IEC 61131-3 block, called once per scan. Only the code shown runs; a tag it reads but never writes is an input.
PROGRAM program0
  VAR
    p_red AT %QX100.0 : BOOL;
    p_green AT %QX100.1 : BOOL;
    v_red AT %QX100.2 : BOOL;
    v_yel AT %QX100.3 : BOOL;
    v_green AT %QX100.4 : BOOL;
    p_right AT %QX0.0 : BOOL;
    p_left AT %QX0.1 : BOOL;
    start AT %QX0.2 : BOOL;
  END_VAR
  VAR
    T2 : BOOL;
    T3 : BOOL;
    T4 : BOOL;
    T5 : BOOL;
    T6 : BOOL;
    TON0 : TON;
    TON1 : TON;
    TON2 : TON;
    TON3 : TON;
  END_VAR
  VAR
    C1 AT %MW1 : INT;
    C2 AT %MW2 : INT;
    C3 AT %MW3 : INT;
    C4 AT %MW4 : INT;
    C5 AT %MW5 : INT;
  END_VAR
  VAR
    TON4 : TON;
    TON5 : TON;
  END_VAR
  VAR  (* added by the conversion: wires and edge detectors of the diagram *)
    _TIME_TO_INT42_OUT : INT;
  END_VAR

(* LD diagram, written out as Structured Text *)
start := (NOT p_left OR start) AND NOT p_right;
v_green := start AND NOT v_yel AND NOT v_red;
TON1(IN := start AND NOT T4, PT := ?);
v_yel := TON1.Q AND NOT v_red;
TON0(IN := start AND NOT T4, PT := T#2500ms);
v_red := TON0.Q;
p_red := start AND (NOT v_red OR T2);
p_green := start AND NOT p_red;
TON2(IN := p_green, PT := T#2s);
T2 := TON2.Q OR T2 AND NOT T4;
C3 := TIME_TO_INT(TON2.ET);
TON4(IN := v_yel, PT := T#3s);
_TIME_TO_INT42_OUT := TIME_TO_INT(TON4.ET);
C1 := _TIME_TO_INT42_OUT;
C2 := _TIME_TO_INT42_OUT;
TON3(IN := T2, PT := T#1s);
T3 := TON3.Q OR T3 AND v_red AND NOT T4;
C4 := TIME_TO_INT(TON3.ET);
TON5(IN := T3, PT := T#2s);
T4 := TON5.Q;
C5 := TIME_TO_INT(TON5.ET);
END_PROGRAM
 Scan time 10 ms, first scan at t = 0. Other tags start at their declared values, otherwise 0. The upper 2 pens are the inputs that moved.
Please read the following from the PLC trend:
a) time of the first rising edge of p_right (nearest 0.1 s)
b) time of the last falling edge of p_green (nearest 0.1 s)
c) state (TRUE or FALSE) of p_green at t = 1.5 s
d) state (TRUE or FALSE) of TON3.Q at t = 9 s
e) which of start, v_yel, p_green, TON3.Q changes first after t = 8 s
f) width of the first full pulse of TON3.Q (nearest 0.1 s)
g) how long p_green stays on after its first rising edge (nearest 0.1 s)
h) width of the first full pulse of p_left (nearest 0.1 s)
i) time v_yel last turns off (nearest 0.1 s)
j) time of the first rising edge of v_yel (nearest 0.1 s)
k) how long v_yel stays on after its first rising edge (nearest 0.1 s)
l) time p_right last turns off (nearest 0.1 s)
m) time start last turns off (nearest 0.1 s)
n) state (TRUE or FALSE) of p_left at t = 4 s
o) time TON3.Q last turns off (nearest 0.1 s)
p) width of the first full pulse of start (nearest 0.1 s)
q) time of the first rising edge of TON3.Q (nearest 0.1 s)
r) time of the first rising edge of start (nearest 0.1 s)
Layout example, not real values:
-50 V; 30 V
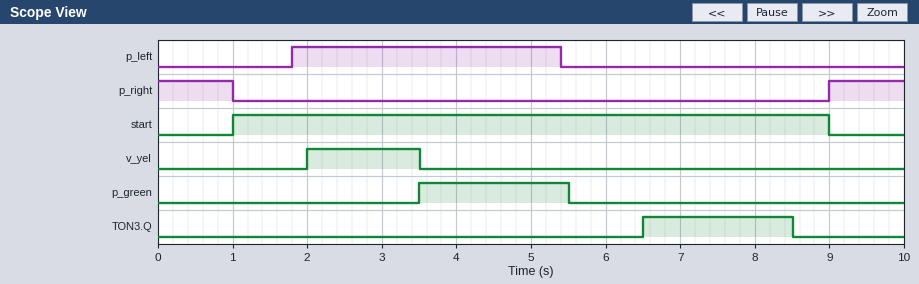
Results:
9.0 s; 5.5 s; FALSE; FALSE; TON3.Q; 2.0 s; 2.0 s; 3.6 s; 3.5 s; 2.0 s; 1.5 s; 1.0 s; 9.0 s; TRUE; 8.5 s; 8.0 s; 6.5 s; 1.0 s
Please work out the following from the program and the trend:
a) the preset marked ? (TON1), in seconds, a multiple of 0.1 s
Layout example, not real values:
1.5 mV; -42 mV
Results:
1.0 s
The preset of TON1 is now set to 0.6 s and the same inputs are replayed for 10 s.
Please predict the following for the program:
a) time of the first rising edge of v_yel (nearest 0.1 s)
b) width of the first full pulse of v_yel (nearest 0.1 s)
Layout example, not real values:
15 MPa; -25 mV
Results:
1.6 s; 1.9 s
